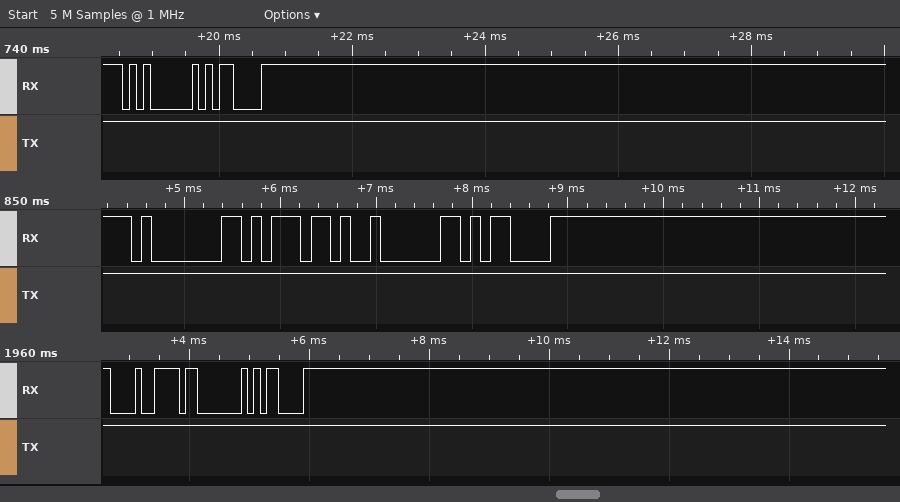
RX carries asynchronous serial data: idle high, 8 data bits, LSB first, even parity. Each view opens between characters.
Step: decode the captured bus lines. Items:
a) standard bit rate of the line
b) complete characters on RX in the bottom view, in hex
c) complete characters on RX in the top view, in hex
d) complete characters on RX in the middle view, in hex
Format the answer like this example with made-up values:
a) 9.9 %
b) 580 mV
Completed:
a) 9600 baud
b) C8, 03, 0D
c) 05, 0D
d) 01, DD, 02, 0D
